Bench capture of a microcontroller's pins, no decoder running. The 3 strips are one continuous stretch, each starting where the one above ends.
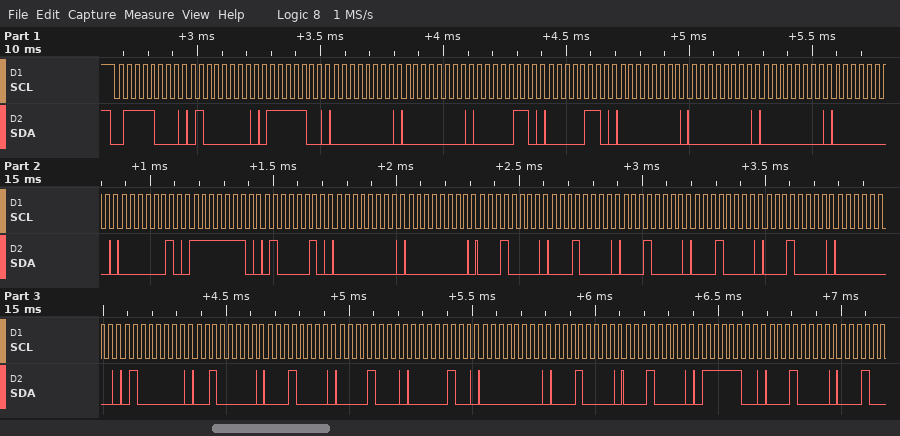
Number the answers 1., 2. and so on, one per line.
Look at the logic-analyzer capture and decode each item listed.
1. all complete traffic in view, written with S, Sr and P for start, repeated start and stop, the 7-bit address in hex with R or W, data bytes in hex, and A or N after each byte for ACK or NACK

1. S 3CW A 40 A 7C A 00 A 00 A 06 A 06 A 00 A 00 A 00 A 00 A 02 A FE A 42 A 00 A 00 A 10 A 10 A 10 A 10 A 10 A 00 A 40 A 20 A 10 A 08 A 04 A 00 A 10 A 10 A 7C A 10 A
